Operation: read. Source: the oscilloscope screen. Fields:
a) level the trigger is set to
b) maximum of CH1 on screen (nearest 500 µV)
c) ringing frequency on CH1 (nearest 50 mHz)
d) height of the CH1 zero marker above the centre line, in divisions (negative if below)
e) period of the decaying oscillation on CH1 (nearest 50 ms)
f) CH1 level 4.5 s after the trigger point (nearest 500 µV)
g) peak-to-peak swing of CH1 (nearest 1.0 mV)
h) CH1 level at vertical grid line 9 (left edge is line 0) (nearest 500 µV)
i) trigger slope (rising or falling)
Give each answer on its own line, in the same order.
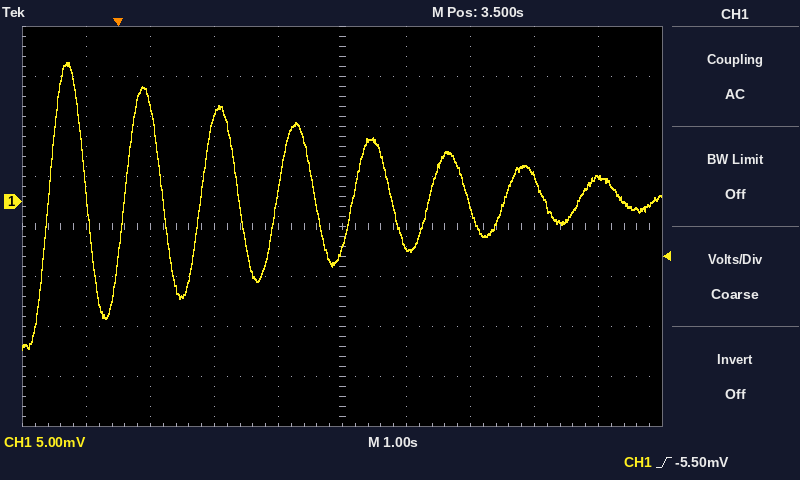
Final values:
-5.50 mV
14.0 mV
850 mHz
+0.5 div
1.20 s
-4.5 mV
29.0 mV
2.5 mV
rising
